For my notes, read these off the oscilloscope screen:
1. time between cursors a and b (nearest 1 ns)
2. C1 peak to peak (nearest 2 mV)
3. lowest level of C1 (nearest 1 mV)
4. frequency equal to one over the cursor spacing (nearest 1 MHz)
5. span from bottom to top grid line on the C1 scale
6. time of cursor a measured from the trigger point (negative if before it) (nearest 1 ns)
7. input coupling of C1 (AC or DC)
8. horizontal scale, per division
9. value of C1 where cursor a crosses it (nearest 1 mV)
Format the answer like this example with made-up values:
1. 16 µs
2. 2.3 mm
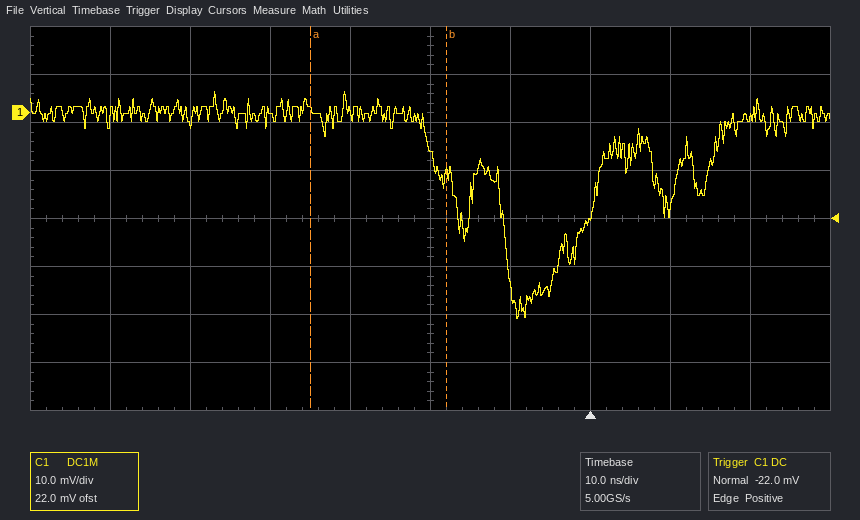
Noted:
1. 17 ns
2. 48 mV
3. -43 mV
4. 59 MHz
5. 80 mV
6. -35 ns
7. DC
8. 10 ns
9. 1 mV
